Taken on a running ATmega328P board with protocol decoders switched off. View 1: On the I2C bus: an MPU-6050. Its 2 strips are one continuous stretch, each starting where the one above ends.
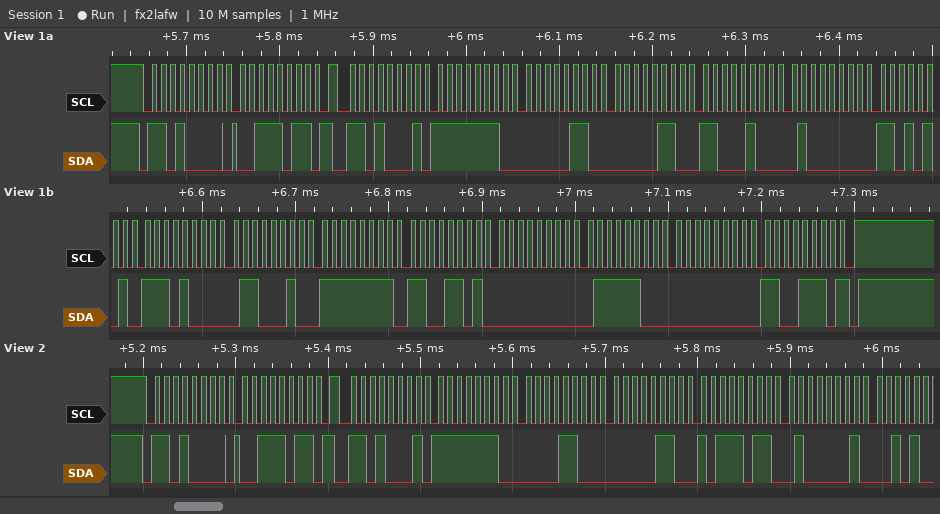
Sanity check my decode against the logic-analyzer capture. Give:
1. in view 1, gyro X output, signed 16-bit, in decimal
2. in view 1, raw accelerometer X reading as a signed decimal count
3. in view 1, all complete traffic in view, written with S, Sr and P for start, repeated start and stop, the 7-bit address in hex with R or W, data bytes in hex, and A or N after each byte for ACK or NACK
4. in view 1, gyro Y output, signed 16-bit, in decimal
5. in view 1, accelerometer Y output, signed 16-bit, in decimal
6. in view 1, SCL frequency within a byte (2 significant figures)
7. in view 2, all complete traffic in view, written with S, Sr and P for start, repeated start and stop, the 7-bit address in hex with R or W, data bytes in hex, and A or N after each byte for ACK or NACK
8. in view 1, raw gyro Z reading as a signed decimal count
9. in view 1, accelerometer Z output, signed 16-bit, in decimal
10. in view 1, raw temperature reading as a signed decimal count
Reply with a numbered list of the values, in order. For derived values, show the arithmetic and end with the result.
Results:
1. 0xFFCD = -51
2. 0xFE06 = -506
3. S 68W A 3B A Sr 68R A FE A 06 A 06 A C4 A 40 A D5 A E8 A 62 A FF A CD A 00 A 7C A 00 A CE N P
4. 0x007C = 124
5. 0x06C4 = 1732
6. 100 kHz
7. S 68W A 3B A Sr 68R A FE A 0C A 06 A BB A 41 A
8. 0x00CE = 206
9. 0x40D5 = 16597
10. 0xE862 = -6046
